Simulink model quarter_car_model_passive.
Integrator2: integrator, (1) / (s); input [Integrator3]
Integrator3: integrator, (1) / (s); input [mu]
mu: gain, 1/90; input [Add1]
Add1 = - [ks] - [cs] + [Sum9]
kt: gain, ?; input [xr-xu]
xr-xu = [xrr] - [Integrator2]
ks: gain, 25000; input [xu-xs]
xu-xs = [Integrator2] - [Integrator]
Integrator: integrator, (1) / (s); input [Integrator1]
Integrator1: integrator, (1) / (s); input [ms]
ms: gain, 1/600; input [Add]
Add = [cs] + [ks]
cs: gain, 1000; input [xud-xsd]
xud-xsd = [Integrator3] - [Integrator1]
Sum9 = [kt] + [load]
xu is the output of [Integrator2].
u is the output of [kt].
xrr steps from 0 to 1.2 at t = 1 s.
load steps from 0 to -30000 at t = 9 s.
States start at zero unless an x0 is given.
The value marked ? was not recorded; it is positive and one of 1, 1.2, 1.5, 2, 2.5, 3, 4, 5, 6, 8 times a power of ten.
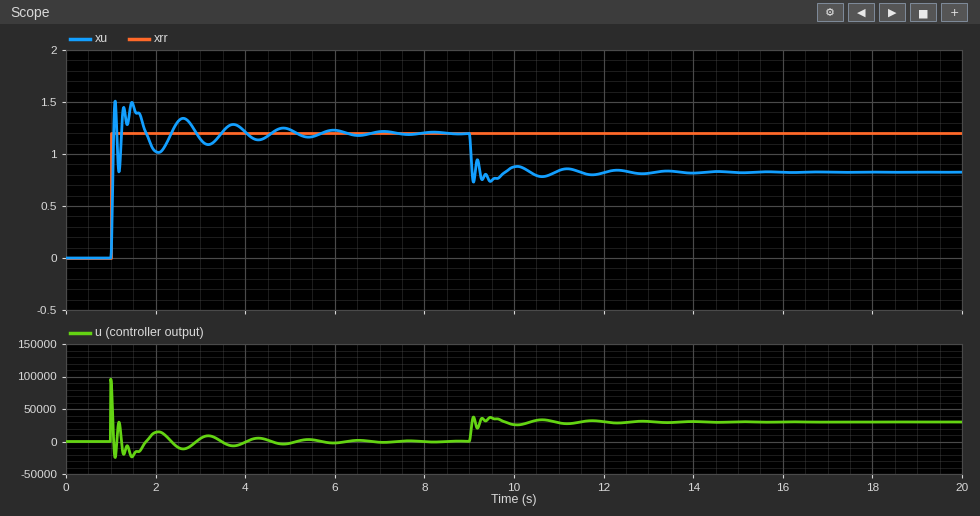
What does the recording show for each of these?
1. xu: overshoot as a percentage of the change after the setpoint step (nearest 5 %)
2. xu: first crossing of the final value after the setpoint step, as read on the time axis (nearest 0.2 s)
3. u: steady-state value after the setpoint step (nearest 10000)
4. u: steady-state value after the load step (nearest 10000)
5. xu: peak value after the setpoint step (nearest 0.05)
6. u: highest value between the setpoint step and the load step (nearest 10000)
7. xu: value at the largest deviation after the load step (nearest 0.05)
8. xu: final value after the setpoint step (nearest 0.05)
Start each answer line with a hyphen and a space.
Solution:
- 25 %
- 1.0 s
- 0
- 30000
- 1.50
- 100000
- 0.75
- 1.20
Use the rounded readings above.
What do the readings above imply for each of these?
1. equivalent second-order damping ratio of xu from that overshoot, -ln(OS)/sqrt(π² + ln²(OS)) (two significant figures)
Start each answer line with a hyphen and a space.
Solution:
- 0.40
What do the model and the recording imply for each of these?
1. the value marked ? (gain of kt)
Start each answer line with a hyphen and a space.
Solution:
- 80000
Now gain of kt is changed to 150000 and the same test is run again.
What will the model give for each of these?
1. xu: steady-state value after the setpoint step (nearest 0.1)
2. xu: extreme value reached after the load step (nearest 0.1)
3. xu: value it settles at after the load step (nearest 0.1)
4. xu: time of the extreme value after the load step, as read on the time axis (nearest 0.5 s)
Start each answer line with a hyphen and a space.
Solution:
- 1.2
- 0.9
- 1.0
- 9.0 s
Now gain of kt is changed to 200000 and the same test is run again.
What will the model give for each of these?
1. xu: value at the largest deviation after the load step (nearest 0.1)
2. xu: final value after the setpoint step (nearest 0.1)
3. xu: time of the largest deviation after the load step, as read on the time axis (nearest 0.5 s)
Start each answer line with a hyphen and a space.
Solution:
- 1.0
- 1.2
- 9.0 s
